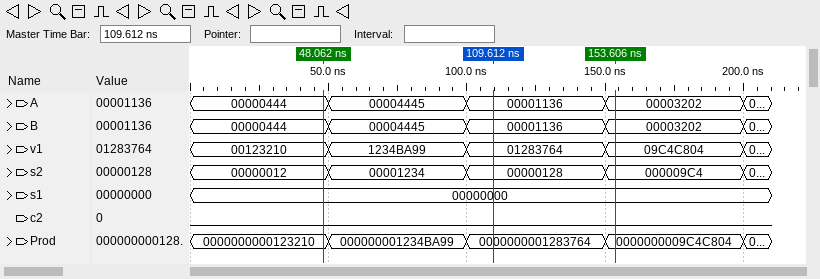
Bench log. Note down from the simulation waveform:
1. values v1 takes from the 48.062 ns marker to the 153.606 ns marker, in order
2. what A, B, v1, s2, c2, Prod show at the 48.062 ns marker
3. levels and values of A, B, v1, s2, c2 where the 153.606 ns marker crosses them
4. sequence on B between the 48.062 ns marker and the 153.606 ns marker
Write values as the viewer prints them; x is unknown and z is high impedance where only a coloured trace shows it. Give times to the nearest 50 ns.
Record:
00123210, 1234BA99, 01283764, 09C4C804
A=00000444, B=00000444, v1=00123210, s2=00000012, c2=0, Prod=0000000000123210
A=00003202, B=00003202, v1=09C4C804, s2=000009C4, c2=0
00000444, 00004445, 00001136, 00003202
